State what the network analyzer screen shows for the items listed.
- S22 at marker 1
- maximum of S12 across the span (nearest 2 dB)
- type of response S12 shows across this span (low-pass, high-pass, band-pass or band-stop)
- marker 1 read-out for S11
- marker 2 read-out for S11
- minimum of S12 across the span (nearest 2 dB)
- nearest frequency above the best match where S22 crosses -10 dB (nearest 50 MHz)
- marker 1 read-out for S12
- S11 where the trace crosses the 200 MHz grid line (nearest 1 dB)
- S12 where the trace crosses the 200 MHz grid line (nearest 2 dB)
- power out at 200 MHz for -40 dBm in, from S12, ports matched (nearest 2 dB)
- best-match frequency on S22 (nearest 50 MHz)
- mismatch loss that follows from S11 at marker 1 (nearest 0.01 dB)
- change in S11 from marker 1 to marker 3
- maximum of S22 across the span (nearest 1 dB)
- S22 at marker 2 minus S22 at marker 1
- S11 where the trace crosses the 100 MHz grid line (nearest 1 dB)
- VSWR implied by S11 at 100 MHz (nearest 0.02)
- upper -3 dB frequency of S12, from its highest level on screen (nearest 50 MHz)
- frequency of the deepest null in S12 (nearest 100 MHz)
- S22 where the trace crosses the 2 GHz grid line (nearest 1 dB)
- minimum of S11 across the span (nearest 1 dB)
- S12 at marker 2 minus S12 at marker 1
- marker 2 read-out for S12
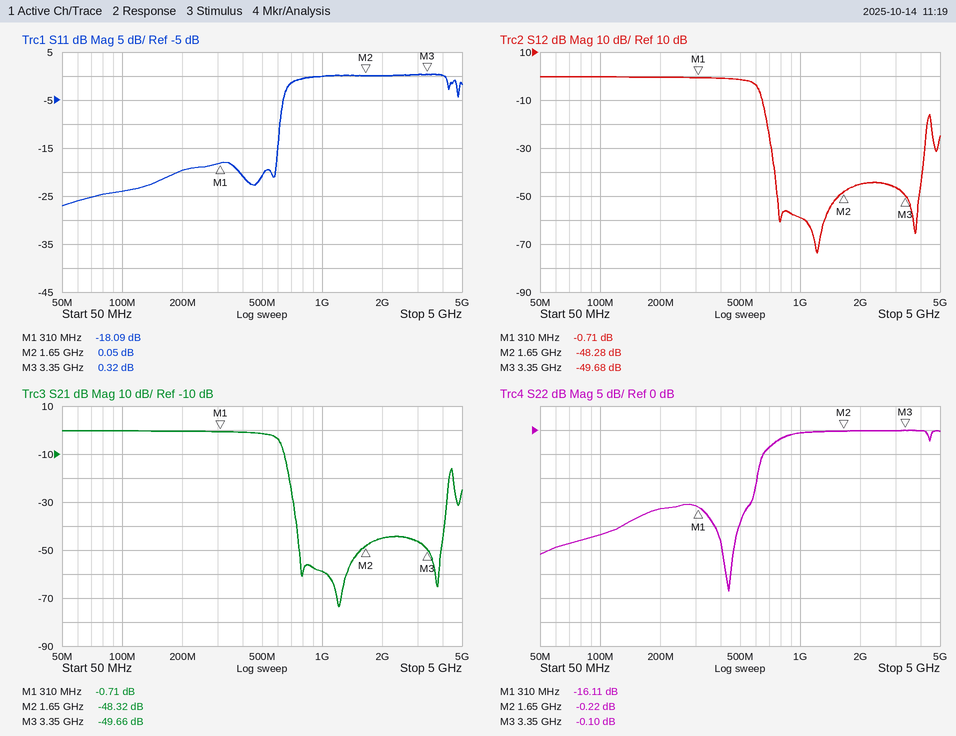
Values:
-16.11 dB
0 dB
low-pass
-18.09 dB
0.05 dB
-74 dB
600 MHz
-0.71 dB
-20 dB
0 dB
-40 dBm
450 MHz
0.07 dB
18.41 dB
0 dB
15.89 dB
-24 dB
1.14
600 MHz
1.2 GHz
0 dB
-27 dB
-47.57 dB
-48.28 dB
